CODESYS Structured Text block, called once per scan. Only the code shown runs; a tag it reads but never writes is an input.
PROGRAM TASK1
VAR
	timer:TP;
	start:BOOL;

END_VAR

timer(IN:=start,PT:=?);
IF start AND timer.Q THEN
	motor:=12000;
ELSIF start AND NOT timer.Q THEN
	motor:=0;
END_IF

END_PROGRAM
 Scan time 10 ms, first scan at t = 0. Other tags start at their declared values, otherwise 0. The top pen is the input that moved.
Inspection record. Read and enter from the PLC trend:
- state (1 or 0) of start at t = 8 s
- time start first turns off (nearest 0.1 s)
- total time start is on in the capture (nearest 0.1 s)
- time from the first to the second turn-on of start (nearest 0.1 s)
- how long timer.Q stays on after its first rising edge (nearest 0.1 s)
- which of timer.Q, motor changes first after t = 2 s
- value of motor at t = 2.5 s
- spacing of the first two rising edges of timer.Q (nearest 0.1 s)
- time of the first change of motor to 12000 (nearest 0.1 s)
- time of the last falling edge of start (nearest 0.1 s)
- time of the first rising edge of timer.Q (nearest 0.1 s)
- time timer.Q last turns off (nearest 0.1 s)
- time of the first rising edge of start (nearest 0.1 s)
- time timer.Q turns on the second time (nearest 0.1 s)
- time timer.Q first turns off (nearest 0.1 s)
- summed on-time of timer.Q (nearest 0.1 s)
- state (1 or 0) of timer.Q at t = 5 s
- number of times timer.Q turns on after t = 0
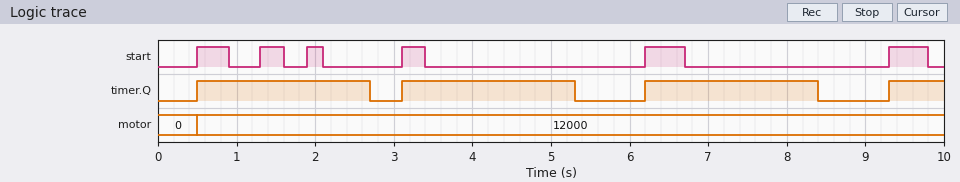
0
0.9 s
2.2 s
0.8 s
2.2 s
timer.Q
12000
2.6 s
0.5 s
9.8 s
0.5 s
8.4 s
0.5 s
3.1 s
2.7 s
7.3 s
1
4
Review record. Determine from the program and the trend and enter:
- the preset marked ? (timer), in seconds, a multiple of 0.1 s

2.2 s
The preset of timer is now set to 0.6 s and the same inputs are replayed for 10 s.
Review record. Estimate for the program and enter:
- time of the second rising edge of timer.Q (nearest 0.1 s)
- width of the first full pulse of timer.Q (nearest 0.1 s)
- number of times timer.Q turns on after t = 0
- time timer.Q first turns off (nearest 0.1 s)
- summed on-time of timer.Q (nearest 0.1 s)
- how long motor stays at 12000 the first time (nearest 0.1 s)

1.3 s
0.6 s
5
1.1 s
3.0 s
1.4 s
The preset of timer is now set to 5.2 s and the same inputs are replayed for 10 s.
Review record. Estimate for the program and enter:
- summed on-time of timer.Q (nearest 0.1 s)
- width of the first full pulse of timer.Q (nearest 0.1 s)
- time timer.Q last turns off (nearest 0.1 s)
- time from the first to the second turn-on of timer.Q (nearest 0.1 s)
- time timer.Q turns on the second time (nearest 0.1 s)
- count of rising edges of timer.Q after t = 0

9.0 s
5.2 s
5.7 s
5.7 s
6.2 s
2
